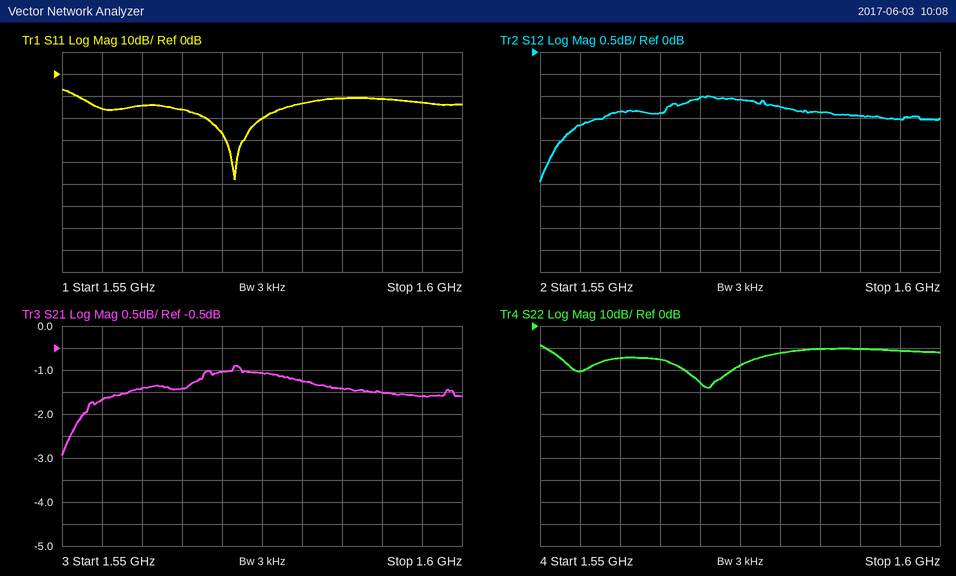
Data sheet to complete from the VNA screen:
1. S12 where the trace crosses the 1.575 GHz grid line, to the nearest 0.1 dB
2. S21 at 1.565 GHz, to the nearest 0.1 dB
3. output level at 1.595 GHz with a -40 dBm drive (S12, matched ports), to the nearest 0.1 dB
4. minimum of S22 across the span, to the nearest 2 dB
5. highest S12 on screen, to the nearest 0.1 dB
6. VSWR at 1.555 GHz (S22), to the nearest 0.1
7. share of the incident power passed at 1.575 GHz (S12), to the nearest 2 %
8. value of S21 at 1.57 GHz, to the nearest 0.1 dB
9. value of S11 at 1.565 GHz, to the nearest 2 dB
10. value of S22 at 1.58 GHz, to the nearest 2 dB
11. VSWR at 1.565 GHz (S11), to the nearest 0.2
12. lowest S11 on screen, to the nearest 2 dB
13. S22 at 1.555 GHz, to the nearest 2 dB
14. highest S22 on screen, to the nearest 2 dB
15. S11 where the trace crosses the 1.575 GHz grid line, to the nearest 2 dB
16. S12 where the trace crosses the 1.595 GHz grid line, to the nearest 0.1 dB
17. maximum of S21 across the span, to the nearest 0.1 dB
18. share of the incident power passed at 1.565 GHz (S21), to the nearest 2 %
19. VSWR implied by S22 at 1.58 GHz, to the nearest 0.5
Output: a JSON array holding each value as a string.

["-1.1 dB", "-1.4 dB", "-41.5 dBm", "-28 dB", "-1.0 dB", "1.2", "78 %", "-1.0 dB", "-16 dB", "-12 dB", "1.4", "-48 dB", "-20 dB", "-8 dB", "-20 dB", "-1.5 dB", "-0.9 dB", "72 %", "1.5"]
